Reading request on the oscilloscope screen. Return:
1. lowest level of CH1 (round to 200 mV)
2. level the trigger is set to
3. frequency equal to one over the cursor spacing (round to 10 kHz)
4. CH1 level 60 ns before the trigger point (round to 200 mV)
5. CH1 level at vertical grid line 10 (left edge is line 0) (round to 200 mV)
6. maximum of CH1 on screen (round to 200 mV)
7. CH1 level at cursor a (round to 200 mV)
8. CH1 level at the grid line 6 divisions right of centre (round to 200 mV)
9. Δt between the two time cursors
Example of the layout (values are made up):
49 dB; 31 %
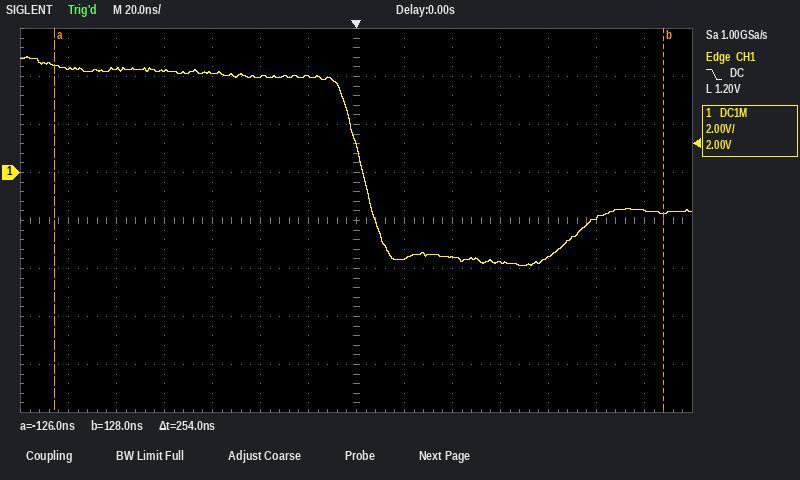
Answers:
-3.8 V; 1.20 V; 3.94 MHz; 4.2 V; -3.8 V; 4.8 V; 4.4 V; -1.6 V; 254 ns
